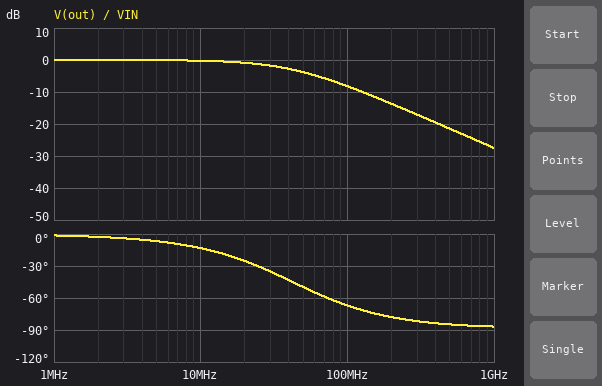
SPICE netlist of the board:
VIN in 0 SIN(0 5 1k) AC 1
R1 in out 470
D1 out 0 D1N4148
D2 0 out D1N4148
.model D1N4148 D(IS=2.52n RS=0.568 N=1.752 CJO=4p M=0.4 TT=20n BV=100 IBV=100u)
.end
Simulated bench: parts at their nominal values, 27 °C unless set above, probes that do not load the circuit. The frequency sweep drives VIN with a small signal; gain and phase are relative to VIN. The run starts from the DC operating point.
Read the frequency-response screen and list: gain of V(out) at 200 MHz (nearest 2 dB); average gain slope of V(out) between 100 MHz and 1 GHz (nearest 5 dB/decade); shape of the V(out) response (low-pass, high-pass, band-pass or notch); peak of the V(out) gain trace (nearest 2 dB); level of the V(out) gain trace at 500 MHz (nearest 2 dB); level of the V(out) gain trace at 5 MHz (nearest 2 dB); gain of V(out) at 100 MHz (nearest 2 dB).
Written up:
-14 dB
-20 dB/decade
low-pass
0 dB
-22 dB
0 dB
-8 dB
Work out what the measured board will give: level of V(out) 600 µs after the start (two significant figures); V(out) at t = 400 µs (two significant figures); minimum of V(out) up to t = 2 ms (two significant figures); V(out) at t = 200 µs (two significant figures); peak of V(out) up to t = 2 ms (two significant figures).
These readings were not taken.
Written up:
-660 mV
660 mV
-690 mV
690 mV
690 mV
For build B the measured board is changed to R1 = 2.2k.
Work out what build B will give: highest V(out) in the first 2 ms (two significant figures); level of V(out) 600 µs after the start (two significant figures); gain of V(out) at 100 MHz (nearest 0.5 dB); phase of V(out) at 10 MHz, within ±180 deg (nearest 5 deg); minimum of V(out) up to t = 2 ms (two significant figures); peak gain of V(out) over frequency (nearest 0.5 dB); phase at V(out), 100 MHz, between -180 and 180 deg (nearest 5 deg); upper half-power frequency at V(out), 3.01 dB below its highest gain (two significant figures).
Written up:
620 mV
-590 mV
-21.0 dB
-50 deg
-620 mV
0 dB
-85 deg
9.0 MHz
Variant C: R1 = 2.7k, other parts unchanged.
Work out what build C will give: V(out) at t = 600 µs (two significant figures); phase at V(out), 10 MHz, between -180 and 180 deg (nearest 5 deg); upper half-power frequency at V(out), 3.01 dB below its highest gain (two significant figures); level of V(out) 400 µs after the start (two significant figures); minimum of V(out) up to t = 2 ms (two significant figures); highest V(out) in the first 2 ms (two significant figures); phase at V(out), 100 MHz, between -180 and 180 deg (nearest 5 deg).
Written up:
-580 mV
-55 deg
7.4 MHz
580 mV
-610 mV
610 mV
-85 deg
